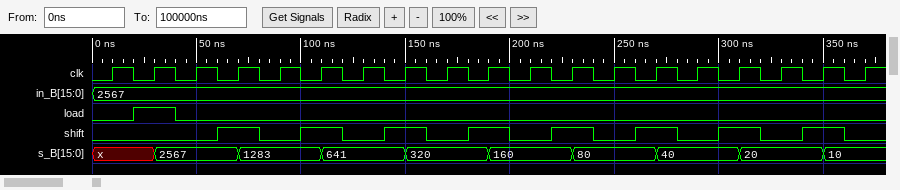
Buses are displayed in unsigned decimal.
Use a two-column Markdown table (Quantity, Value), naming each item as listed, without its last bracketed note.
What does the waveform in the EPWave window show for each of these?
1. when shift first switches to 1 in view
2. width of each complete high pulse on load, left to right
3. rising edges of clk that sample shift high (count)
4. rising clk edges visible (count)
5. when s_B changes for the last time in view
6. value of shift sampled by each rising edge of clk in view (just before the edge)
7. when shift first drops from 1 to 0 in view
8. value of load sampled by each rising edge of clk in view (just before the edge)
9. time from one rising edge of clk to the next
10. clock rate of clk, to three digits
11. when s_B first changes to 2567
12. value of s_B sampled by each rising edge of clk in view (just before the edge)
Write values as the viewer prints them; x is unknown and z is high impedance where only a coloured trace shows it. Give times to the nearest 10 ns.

| Quantity | Value |
|---|---|
| when shift first switches to 1 in view | 60 ns |
| width of each complete high pulse on load, left to right | 20 ns |
| rising edges of clk that sample shift high | 8 |
| rising clk edges visible | 19 |
| when s_B changes for the last time in view | 350 ns |
| value of shift sampled by each rising edge of clk in view | 0 0 0 1 0 1 0 1 0 1 0 1 0 1 0 1 0 1 0 |
| when shift first drops from 1 to 0 in view | 80 ns |
| value of load sampled by each rising edge of clk in view | 0 1 0 0 0 0 0 0 0 0 0 0 0 0 0 0 0 0 0 |
| time from one rising edge of clk to the next | 20 ns |
| clock rate of clk, to three digits | 50.0 MHz |
| when s_B first changes to 2567 | 30 ns |
| value of s_B sampled by each rising edge of clk in view | x, x, 2567, 2567, 1283, 1283, 641, 641, 320, 320, 160, 160, 80, 80, 40, 40, 20, 20, 10 |
